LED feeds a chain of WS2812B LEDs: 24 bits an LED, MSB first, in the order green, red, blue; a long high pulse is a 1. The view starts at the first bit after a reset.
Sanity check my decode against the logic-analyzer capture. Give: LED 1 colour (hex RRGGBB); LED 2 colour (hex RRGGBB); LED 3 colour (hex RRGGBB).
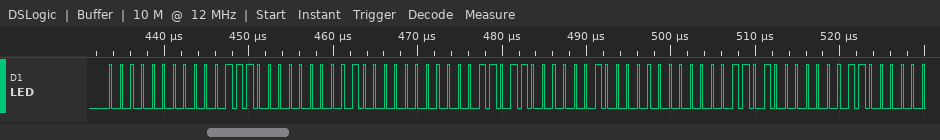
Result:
#1C0001
#1B0002
#1A0003
